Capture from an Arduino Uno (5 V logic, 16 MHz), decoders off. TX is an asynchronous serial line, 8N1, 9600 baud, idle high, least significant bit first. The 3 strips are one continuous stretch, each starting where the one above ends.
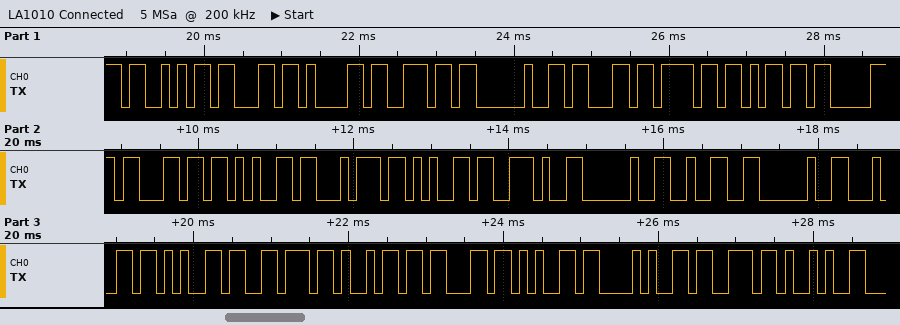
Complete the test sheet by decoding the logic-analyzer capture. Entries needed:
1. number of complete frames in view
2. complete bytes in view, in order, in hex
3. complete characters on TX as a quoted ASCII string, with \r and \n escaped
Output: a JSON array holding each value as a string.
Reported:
["26", "53 63 61 6E 20 63 6F 6D 70 6C 65 74 65 2E 20 32 20 64 65 76 69 63 65 28 73 29", "\"Scan complete. 2 device(s)\""]
